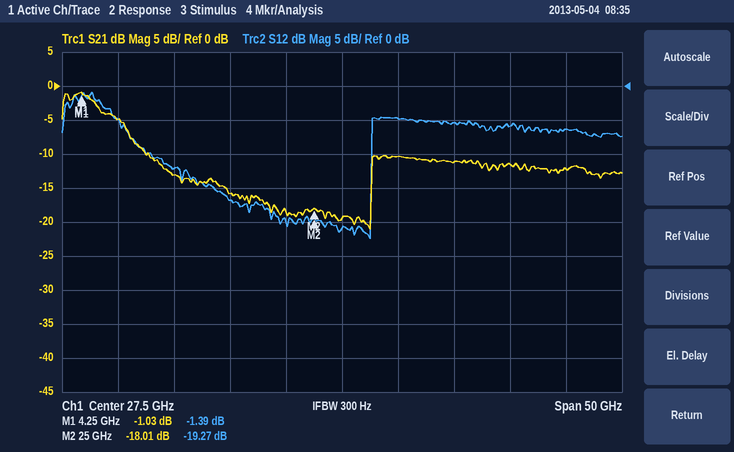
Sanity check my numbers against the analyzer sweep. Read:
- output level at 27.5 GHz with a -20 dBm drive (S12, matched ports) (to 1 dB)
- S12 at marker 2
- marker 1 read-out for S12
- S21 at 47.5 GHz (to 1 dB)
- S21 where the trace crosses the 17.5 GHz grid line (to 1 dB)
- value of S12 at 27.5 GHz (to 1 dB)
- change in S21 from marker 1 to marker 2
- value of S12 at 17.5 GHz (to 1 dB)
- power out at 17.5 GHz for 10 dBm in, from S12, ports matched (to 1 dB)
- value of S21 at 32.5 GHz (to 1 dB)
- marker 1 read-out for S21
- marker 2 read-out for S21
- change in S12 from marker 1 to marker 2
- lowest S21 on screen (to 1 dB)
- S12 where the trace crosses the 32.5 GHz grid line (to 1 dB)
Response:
-41 dBm
-19.27 dB
-1.39 dB
-12 dB
-16 dB
-21 dB
-16.98 dB
-17 dB
-7 dBm
-10 dB
-1.03 dB
-18.01 dB
-17.88 dB
-21 dB
-5 dB
